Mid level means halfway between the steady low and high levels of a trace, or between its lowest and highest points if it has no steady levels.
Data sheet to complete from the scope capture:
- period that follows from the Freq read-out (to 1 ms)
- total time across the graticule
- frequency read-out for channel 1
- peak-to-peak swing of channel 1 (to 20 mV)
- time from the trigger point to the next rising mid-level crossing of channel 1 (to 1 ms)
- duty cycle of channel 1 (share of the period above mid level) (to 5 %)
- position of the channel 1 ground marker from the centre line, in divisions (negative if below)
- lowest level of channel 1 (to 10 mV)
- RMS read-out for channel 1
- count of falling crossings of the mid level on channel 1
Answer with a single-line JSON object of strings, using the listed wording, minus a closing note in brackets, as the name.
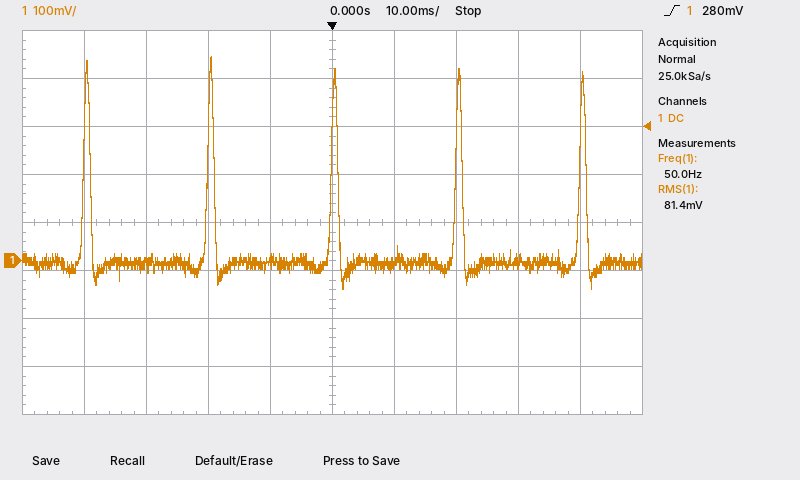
{"period that follows from the Freq read-out": "20 ms", "total time across the graticule": "100 ms", "frequency read-out for channel 1": "50.0 Hz", "peak-to-peak swing of channel 1": "480 mV", "time from the trigger point to the next rising mid-level crossing of channel 1": "20 ms", "duty cycle of channel 1 (share of the period above mid level)": "5 %", "position of the channel 1 ground marker from the centre line, in divisions": "-0.8 div", "lowest level of channel 1": "-60 mV", "RMS read-out for channel 1": "81.4 mV", "count of falling crossings of the mid level on channel 1": "5"}
